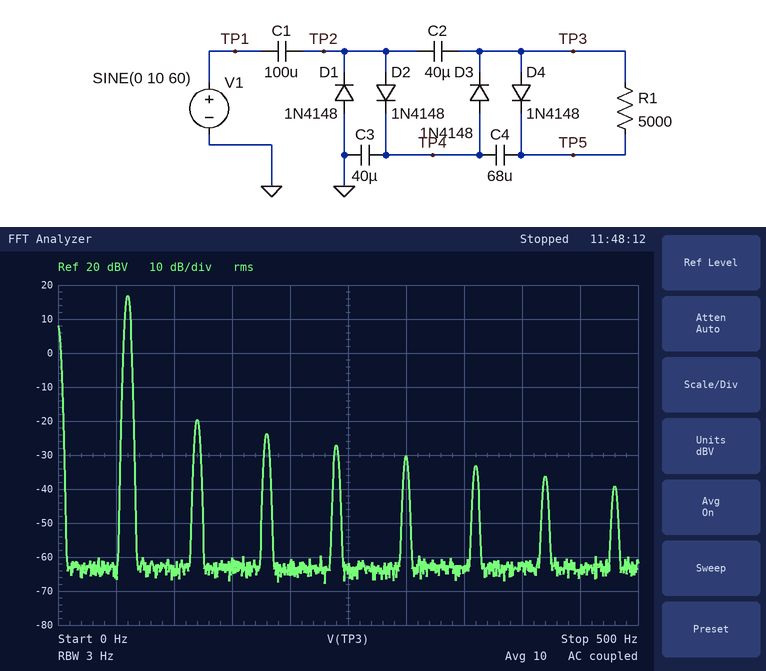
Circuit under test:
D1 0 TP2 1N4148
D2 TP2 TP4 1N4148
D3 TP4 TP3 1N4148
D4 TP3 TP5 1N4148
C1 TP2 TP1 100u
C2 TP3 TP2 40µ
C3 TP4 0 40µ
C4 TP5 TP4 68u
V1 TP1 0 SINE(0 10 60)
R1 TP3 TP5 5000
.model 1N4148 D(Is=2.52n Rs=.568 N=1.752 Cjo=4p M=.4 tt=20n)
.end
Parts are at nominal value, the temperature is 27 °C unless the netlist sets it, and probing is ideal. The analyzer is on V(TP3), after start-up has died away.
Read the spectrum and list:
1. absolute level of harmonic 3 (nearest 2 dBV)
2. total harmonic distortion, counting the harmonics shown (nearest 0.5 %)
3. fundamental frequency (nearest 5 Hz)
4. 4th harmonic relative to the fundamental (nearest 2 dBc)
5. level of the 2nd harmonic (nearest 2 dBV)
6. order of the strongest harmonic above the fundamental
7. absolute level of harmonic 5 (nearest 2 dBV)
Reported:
-24 dBV
2.0 %
60 Hz
-44 dBc
-20 dBV
2
-30 dBV
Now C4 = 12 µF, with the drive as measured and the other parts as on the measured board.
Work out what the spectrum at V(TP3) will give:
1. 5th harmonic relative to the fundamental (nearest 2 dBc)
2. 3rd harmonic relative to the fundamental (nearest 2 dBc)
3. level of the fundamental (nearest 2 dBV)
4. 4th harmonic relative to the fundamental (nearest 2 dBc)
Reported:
-50 dBc
-42 dBc
16 dBV
-46 dBc
